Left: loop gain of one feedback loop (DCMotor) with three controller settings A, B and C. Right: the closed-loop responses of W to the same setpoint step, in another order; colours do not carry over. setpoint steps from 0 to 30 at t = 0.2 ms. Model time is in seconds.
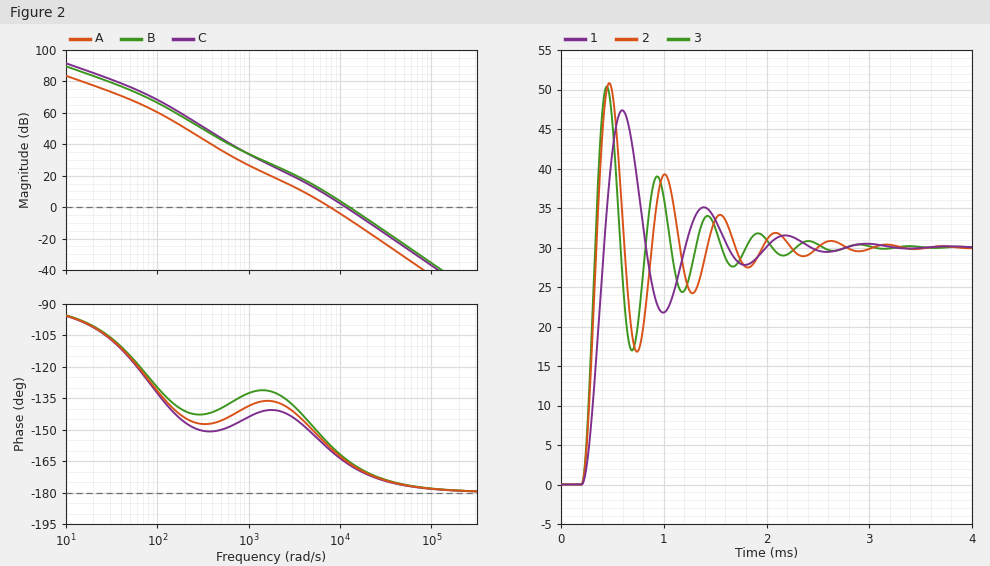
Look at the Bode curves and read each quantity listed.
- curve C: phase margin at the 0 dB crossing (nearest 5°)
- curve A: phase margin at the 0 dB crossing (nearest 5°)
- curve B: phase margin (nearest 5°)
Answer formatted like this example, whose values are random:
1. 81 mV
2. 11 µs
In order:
1. 15°
2. 20°
3. 15°
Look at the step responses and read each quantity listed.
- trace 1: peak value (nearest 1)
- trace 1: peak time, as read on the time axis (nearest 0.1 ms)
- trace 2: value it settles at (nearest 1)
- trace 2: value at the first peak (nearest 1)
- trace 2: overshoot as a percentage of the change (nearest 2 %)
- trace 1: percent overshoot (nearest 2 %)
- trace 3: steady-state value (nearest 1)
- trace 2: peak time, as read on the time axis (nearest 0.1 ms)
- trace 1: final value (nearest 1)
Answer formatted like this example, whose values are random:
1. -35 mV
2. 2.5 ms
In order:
1. 47
2. 0.6 ms
3. 30
4. 51
5. 70 %
6. 58 %
7. 30
8. 0.5 ms
9. 30
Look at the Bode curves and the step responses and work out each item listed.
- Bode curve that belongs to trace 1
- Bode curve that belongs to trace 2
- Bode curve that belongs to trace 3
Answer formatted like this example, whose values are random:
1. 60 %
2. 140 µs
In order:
1. A
2. C
3. B
